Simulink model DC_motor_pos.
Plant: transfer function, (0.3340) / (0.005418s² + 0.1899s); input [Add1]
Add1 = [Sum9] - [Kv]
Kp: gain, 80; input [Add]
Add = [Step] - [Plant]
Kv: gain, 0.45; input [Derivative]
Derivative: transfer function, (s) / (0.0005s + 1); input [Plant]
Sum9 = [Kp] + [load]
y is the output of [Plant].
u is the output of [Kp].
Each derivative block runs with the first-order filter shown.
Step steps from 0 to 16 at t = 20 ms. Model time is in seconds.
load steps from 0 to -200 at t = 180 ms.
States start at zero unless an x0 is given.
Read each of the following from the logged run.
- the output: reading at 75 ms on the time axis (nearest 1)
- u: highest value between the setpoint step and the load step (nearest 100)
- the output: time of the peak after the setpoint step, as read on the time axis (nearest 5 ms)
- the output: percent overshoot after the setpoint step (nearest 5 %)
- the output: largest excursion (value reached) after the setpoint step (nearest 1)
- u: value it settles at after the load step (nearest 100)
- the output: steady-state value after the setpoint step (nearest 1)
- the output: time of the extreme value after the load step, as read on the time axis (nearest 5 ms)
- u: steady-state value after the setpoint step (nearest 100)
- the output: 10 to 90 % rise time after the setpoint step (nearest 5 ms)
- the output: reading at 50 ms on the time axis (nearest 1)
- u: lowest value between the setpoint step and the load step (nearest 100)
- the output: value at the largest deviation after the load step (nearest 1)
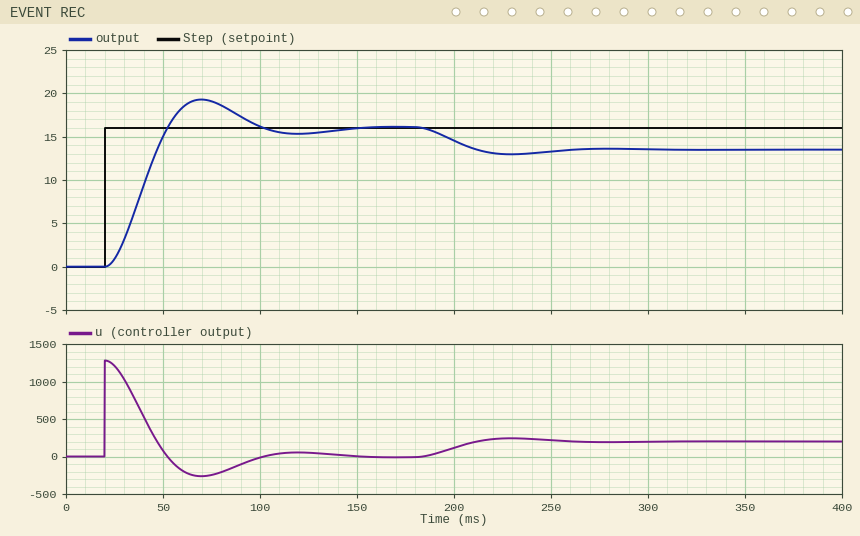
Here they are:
19
1300
70 ms
20 %
19
200
16
230 ms
0
20 ms
15
-300
13
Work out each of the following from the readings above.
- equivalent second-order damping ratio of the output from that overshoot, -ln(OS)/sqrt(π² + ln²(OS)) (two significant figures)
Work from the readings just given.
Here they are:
0.46
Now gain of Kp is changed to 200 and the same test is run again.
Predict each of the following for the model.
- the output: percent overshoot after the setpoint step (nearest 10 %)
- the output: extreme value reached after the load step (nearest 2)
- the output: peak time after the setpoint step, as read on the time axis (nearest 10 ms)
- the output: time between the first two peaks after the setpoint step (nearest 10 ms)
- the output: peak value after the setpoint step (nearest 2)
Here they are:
40 %
14
50 ms
60 ms
22
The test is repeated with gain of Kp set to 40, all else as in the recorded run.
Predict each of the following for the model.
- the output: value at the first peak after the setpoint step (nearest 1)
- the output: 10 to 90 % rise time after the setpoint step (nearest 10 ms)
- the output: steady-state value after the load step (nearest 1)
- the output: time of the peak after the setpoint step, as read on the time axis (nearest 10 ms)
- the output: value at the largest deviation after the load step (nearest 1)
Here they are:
17
40 ms
11
100 ms
11
